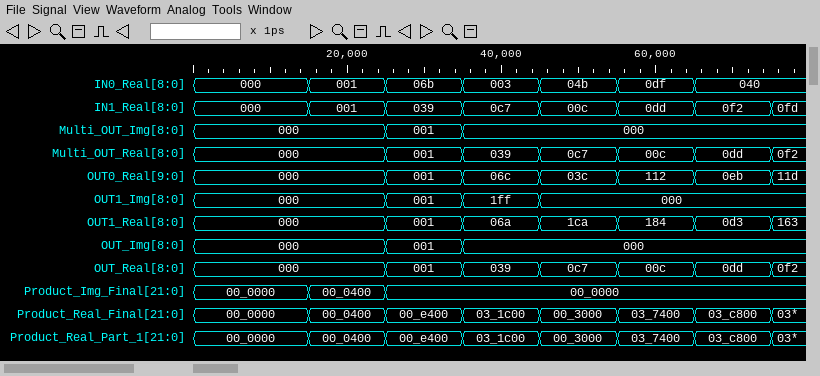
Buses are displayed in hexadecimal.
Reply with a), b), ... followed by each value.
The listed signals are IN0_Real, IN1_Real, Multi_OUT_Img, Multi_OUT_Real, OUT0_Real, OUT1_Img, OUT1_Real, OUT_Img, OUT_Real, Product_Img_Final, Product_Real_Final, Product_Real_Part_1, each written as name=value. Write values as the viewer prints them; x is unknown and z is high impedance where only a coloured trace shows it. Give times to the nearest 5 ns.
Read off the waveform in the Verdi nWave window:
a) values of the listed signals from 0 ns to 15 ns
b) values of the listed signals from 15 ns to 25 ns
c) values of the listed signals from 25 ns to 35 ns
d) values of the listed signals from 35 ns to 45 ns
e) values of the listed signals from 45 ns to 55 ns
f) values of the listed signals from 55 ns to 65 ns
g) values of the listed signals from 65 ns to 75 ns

a) IN0_Real=000, IN1_Real=000, Multi_OUT_Img=000, Multi_OUT_Real=000, OUT0_Real=000, OUT1_Img=000, OUT1_Real=000, OUT_Img=000, OUT_Real=000, Product_Img_Final=00_0000, Product_Real_Final=00_0000, Product_Real_Part_1=00_0000
b) IN0_Real=001, IN1_Real=001, Multi_OUT_Img=000, Multi_OUT_Real=000, OUT0_Real=000, OUT1_Img=000, OUT1_Real=000, OUT_Img=000, OUT_Real=000, Product_Img_Final=00_0400, Product_Real_Final=00_0400, Product_Real_Part_1=00_0400
c) IN0_Real=06b, IN1_Real=039, Multi_OUT_Img=001, Multi_OUT_Real=001, OUT0_Real=001, OUT1_Img=001, OUT1_Real=001, OUT_Img=001, OUT_Real=001, Product_Img_Final=00_0000, Product_Real_Final=00_e400, Product_Real_Part_1=00_e400
d) IN0_Real=003, IN1_Real=0c7, Multi_OUT_Img=000, Multi_OUT_Real=039, OUT0_Real=06c, OUT1_Img=1ff, OUT1_Real=06a, OUT_Img=000, OUT_Real=039, Product_Img_Final=00_0000, Product_Real_Final=03_1c00, Product_Real_Part_1=03_1c00
e) IN0_Real=04b, IN1_Real=00c, Multi_OUT_Img=000, Multi_OUT_Real=0c7, OUT0_Real=03c, OUT1_Img=000, OUT1_Real=1ca, OUT_Img=000, OUT_Real=0c7, Product_Img_Final=00_0000, Product_Real_Final=00_3000, Product_Real_Part_1=00_3000
f) IN0_Real=0df, IN1_Real=0dd, Multi_OUT_Img=000, Multi_OUT_Real=00c, OUT0_Real=112, OUT1_Img=000, OUT1_Real=184, OUT_Img=000, OUT_Real=00c, Product_Img_Final=00_0000, Product_Real_Final=03_7400, Product_Real_Part_1=03_7400
g) IN0_Real=040, IN1_Real=0f2, Multi_OUT_Img=000, Multi_OUT_Real=0dd, OUT0_Real=0eb, OUT1_Img=000, OUT1_Real=0d3, OUT_Img=000, OUT_Real=0dd, Product_Img_Final=00_0000, Product_Real_Final=03_c800, Product_Real_Part_1=03_c800
